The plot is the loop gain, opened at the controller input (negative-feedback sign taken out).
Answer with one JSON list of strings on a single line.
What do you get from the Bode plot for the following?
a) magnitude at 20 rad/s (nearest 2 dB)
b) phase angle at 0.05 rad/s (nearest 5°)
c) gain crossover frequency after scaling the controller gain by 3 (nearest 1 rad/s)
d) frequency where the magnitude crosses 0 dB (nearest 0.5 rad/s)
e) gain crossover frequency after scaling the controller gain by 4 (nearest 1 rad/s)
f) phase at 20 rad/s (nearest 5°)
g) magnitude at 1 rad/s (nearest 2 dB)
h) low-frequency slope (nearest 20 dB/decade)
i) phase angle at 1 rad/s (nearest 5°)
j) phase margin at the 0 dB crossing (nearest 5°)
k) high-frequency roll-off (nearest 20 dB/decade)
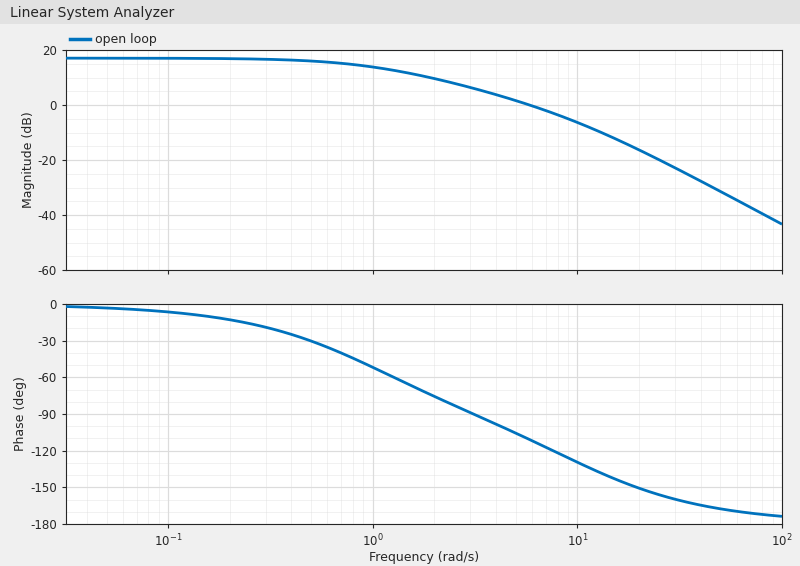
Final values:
["-16 dB", "-5°", "13 rad/s", "6.0 rad/s", "15 rad/s", "-150°", "14 dB", "0 dB/decade", "-50°", "70°", "-40 dB/decade"]
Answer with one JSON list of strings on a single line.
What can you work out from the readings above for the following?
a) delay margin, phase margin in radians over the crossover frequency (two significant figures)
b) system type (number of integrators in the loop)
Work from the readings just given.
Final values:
["0.20 s", "0"]
